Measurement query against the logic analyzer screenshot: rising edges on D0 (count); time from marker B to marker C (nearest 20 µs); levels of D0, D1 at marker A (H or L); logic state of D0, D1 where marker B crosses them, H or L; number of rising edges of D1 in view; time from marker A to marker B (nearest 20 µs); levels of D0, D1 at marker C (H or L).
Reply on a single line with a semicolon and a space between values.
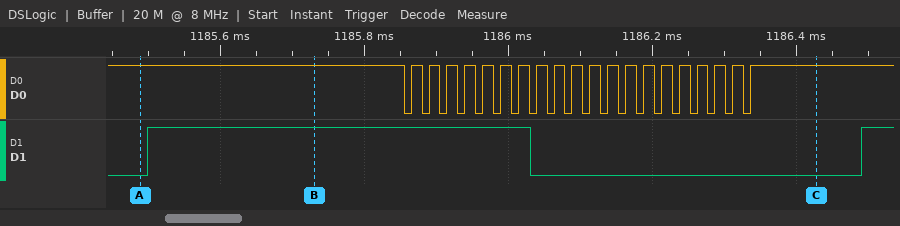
20; 700 µs; D0=H, D1=L; D0=H, D1=H; 2; 240 µs; D0=H, D1=L
